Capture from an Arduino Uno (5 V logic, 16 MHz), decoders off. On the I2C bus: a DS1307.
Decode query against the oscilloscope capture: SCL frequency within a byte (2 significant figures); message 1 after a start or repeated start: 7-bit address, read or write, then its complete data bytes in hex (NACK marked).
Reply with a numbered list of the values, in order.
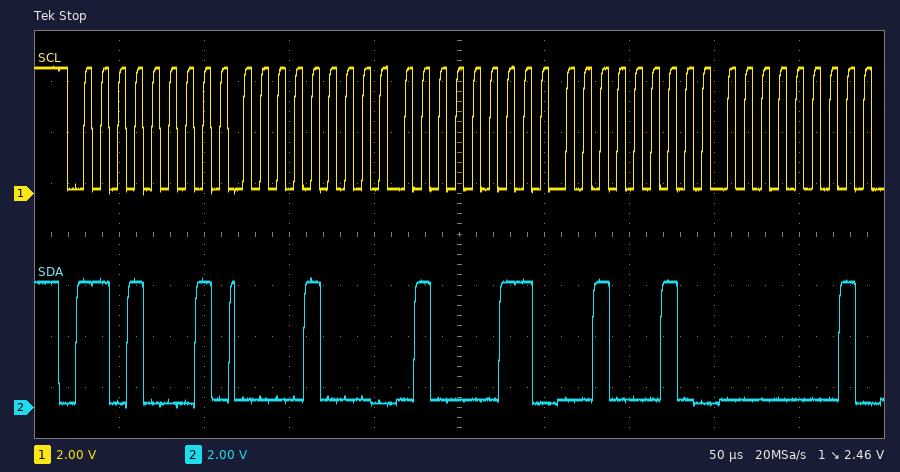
1. 100 kHz
2. 0x68 read: 08 43 22 01
